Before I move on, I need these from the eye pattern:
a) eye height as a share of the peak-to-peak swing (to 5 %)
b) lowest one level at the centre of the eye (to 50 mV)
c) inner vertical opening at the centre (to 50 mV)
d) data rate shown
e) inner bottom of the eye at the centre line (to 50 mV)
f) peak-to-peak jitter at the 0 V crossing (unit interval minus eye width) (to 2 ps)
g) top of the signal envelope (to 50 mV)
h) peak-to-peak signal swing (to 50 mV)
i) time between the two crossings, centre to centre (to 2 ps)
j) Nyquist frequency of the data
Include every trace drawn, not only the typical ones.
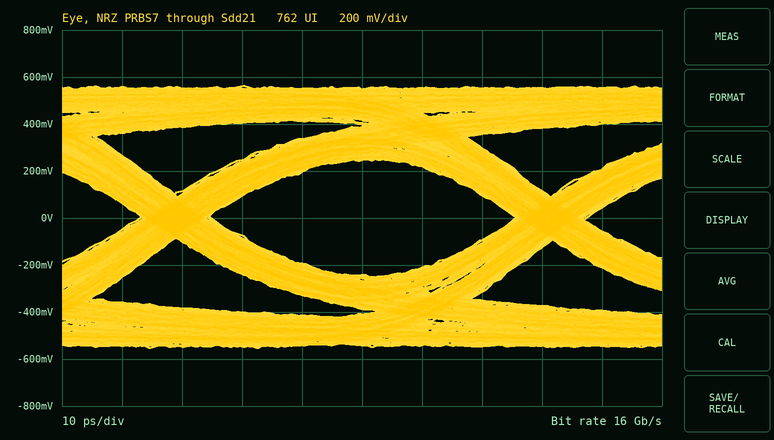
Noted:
45 %
250 mV
500 mV
16 Gb/s
-250 mV
12 ps
550 mV
1.10 V
62 ps
8 GHz
